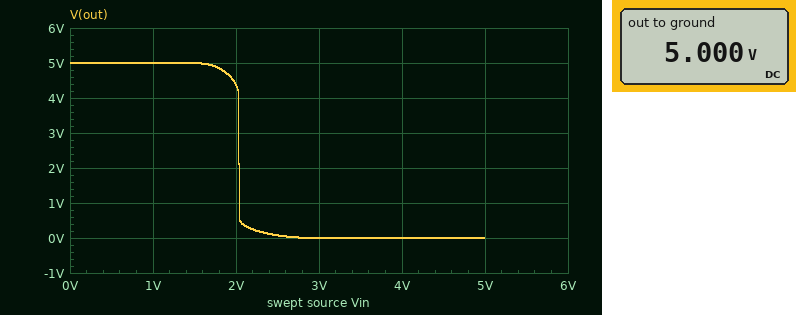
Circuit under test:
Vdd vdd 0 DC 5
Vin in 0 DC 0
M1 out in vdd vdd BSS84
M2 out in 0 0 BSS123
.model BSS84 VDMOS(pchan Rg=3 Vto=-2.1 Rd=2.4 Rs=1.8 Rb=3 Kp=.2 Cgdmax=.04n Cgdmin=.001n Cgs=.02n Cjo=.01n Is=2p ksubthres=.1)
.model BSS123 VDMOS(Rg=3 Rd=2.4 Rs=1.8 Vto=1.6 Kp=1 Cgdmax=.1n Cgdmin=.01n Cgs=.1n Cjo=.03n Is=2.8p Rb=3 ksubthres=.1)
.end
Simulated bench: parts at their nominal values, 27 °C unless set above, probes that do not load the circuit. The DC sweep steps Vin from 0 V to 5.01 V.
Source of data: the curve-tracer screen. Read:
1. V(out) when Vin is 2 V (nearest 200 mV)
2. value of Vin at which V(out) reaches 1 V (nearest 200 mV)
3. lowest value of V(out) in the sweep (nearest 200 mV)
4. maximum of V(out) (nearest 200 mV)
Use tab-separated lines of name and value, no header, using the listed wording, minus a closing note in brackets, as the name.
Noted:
V(out) when Vin is 2 V	4.4 V
value of Vin at which V(out) reaches 1 V	2.0 V
lowest value of V(out) in the sweep	0 V
maximum of V(out)	5.0 V
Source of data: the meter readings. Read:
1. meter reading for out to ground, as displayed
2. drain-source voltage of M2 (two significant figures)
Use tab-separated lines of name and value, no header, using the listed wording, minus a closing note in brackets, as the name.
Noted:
meter reading for out to ground, as displayed	5.000 V
drain-source voltage of M2	5.0 V
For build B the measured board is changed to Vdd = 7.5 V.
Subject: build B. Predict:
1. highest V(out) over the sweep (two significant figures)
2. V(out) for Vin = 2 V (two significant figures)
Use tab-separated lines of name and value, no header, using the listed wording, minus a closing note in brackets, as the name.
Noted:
highest V(out) over the sweep	7.5 V
V(out) for Vin = 2 V	7.2 V
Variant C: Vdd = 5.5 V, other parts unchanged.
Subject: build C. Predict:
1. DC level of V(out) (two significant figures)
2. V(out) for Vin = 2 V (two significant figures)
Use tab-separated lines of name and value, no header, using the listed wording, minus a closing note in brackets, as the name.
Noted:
DC level of V(out)	5.5 V
V(out) for Vin = 2 V	5.1 V
